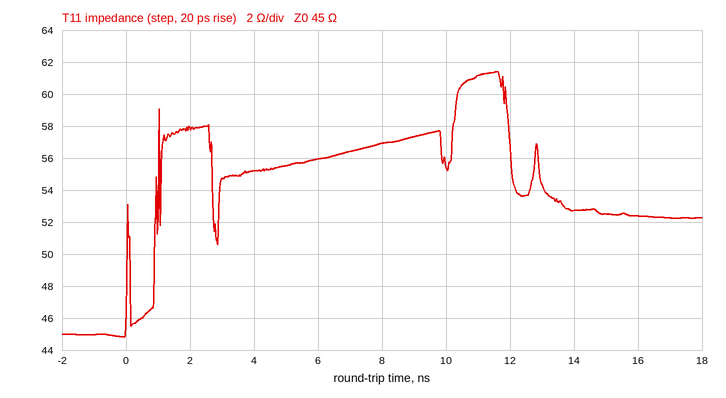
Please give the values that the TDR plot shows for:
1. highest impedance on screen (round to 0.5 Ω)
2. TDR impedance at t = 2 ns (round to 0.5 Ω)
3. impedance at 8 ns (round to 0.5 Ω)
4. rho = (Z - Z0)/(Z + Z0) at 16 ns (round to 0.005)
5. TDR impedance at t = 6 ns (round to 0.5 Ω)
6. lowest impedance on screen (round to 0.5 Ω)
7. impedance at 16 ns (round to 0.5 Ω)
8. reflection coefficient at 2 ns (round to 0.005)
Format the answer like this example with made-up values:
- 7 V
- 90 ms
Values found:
- 61.5 Ω
- 58.0 Ω
- 57.0 Ω
- +0.075
- 56.0 Ω
- 45.0 Ω
- 52.5 Ω
- +0.125
